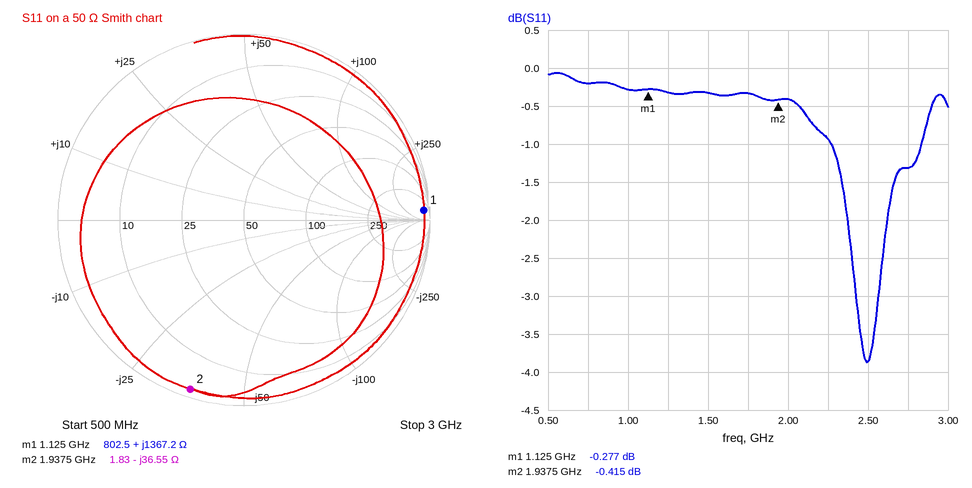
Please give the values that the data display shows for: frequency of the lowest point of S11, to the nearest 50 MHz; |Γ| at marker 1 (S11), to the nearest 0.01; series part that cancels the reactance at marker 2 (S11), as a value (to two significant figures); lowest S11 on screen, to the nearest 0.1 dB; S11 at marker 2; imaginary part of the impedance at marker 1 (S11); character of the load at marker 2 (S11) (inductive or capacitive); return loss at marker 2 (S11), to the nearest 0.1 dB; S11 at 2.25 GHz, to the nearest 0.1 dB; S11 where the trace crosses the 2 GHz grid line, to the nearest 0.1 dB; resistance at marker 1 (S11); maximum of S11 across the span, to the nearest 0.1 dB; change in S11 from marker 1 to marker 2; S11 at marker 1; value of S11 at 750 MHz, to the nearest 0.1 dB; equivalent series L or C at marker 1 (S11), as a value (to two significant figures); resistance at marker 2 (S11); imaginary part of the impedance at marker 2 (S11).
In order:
2.50 GHz
0.97
3.0 nH
-3.9 dB
-0.415 dB
+1367.2 Ω
capacitive
0.4 dB
-0.9 dB
-0.4 dB
802.5 Ω
-0.1 dB
-0.138 dB
-0.277 dB
-0.2 dB
190 nH
1.83 Ω
-36.55 Ω
